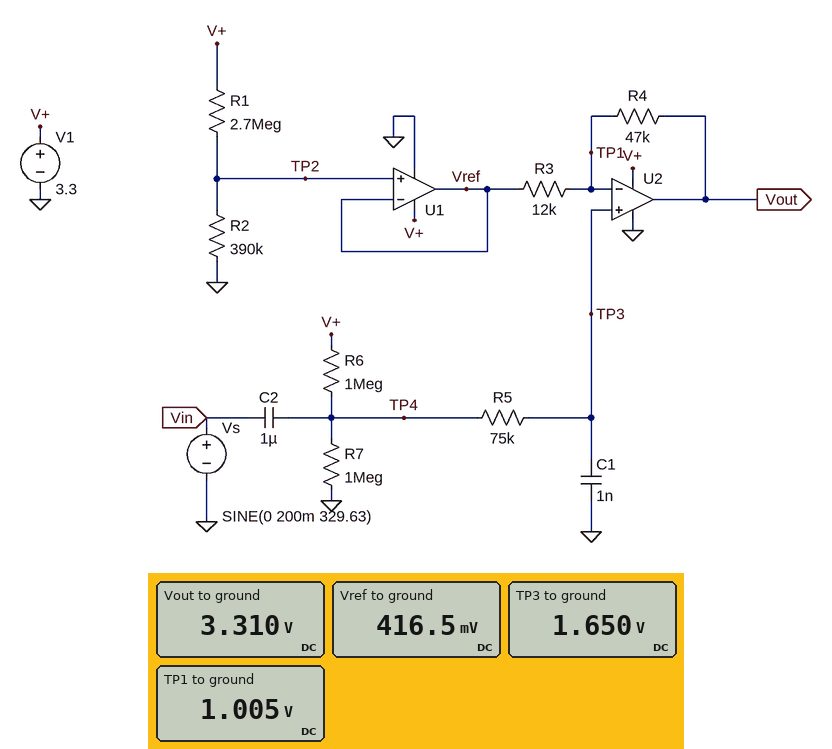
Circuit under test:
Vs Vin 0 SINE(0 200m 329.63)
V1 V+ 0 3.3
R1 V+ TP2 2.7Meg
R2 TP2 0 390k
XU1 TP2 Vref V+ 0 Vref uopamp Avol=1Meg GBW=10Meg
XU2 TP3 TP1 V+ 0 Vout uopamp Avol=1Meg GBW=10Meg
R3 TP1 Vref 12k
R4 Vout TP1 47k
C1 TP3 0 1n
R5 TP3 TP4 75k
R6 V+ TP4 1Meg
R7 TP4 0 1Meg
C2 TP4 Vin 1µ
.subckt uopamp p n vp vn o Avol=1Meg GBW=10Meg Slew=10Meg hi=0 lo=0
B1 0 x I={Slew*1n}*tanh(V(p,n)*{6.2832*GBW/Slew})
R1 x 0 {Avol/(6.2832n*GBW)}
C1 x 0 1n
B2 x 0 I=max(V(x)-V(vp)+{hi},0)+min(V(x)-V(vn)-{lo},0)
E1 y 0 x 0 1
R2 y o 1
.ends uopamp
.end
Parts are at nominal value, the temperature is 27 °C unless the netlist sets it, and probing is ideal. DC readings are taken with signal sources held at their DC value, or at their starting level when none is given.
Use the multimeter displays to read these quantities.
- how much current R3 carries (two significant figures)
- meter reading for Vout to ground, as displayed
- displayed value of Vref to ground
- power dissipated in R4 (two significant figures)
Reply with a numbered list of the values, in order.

1. 49 µA
2. 3.310 V
3. 416.5 mV
4. 110 µW
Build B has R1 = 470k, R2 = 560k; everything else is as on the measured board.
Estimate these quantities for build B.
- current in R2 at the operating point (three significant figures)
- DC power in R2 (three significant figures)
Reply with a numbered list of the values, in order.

1. 3.20 µA
2. 5.75 µW
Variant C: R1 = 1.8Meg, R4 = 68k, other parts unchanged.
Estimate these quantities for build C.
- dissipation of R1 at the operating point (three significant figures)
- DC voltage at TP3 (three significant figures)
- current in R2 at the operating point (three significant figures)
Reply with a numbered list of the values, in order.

1. 4.09 µW
2. 1.65 V
3. 1.51 µA
